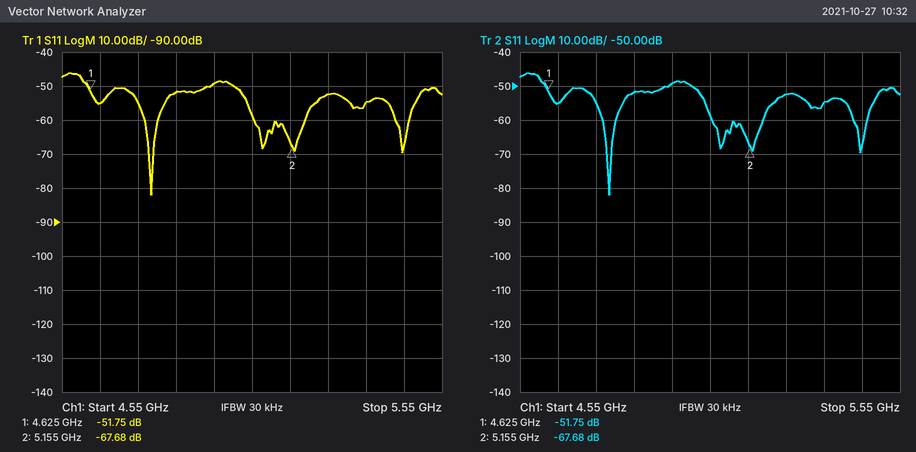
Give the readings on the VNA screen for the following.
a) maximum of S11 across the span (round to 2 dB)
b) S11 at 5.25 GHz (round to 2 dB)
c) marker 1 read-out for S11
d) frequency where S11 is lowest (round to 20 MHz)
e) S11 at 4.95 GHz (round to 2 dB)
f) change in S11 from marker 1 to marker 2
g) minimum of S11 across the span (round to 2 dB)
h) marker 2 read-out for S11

-46 dB
-52 dB
-51.75 dB
4.78 GHz
-50 dB
-15.93 dB
-82 dB
-67.68 dB
